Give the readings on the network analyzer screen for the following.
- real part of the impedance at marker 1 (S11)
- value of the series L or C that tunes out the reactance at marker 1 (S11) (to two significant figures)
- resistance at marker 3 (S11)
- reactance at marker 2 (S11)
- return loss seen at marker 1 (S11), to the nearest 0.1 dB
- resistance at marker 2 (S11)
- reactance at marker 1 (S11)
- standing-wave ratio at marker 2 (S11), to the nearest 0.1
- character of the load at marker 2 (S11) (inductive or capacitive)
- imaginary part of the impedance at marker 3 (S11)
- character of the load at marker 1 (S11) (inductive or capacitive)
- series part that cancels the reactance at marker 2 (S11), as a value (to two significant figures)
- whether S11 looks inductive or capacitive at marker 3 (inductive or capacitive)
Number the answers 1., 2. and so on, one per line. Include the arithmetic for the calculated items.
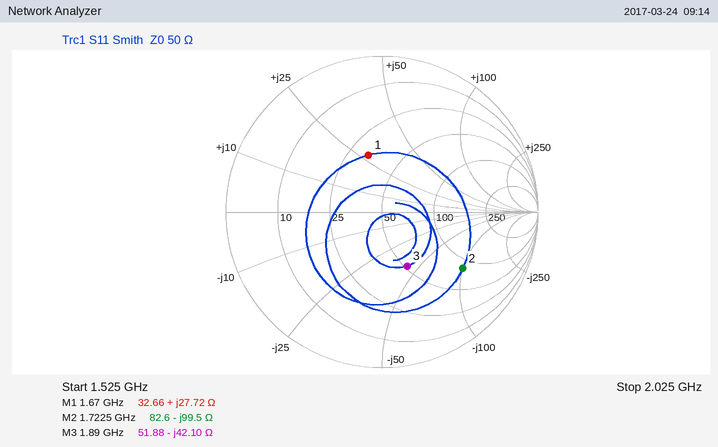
1. 32.66 Ω
2. C = 1/(2π × 1.67 GHz × 27.72 Ω) ≈ 3.4 pF
3. 51.88 Ω
4. -99.5 Ω
5. 8.5 dB
6. 82.6 Ω
7. +27.72 Ω
8. 4.4
9. capacitive
10. -42.10 Ω
11. inductive
12. L = 99.5 Ω/(2π × 1.7225 GHz) ≈ 9.2 nH
13. capacitive
